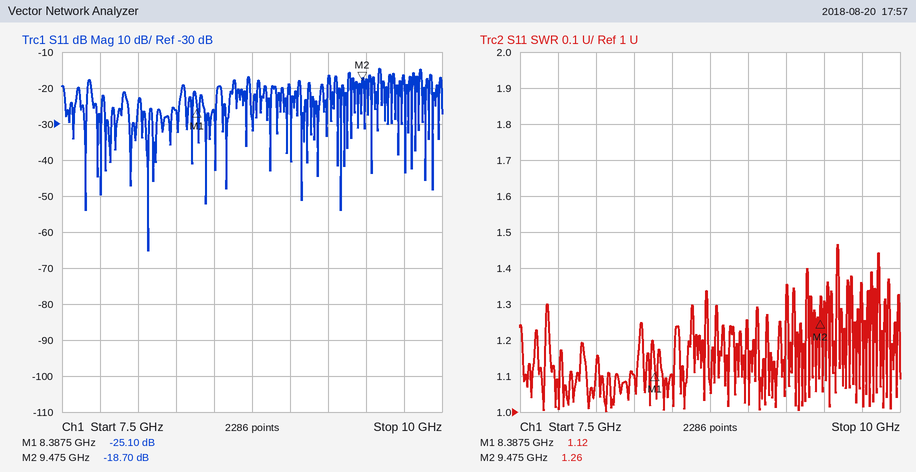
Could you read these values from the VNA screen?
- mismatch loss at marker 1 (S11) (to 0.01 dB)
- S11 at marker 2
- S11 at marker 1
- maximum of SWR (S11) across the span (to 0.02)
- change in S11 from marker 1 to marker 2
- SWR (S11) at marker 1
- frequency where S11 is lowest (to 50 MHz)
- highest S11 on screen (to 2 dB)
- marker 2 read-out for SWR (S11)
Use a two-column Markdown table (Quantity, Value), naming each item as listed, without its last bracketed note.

| Quantity | Value |
|---|---|
| mismatch loss at marker 1 (S11) | 0.01 dB |
| S11 at marker 2 | -18.70 dB |
| S11 at marker 1 | -25.10 dB |
| maximum of SWR (S11) across the span | 1.46 |
| change in S11 from marker 1 to marker 2 | 6.40 dB |
| SWR (S11) at marker 1 | 1.12 |
| frequency where S11 is lowest | 8.05 GHz |
| highest S11 on screen | -14 dB |
| marker 2 read-out for SWR | 1.26 |
